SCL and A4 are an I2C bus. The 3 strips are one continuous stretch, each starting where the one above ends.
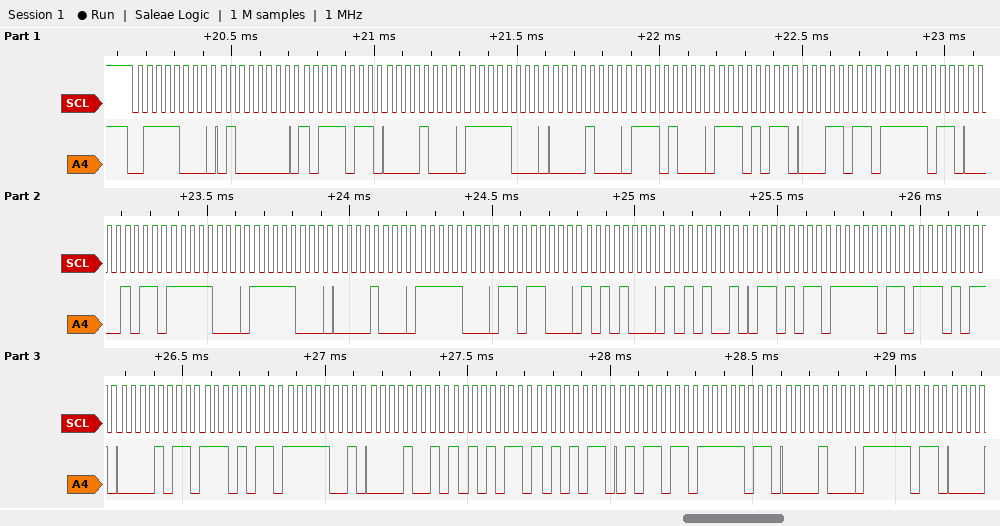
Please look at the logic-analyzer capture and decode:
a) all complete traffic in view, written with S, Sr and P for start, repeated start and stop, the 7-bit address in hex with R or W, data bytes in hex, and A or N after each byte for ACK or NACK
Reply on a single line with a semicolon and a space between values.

S 3CW A 40 A BB A 08 A F8 A 08 A E8 A EB A 1B A FB A 0B A F8 A F8 A 08 A F8 A D8 A A8 A A9 A 6B A FB A EB A 0B A EB A F9 A 09 A AB A AB A 5B A FB A 08 A FB A
